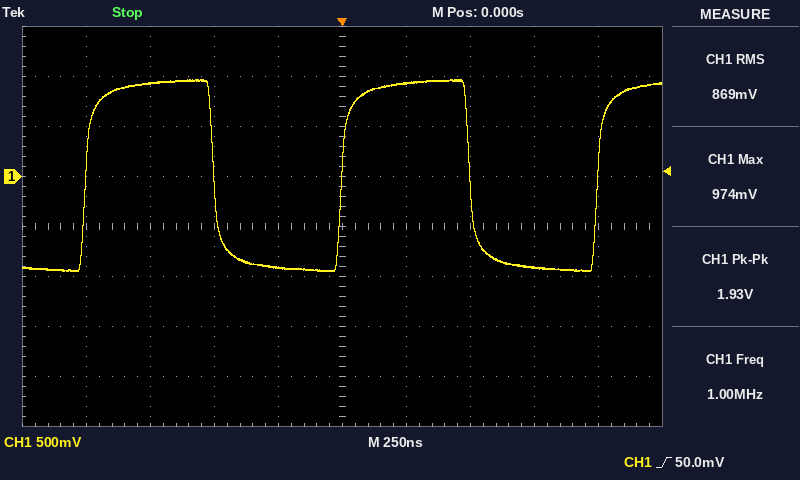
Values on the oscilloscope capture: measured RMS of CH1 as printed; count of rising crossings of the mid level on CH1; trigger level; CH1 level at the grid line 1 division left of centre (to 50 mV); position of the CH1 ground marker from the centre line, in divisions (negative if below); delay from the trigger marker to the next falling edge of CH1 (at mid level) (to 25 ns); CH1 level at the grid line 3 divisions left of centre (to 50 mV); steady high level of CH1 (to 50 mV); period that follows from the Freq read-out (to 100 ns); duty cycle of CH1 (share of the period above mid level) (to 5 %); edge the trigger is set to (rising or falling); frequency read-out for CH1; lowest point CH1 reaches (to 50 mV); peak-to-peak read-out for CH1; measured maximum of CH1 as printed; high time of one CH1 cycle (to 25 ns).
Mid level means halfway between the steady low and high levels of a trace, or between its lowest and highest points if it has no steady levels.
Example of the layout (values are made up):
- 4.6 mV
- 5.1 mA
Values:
- 869 mV
- 3
- 50.0 mV
- -900 mV
- +1.0 div
- 500 ns
- 950 mV
- 950 mV
- 1.0 µs
- 50 %
- rising
- 1.00 MHz
- -950 mV
- 1.93 V
- 974 mV
- 500 ns
